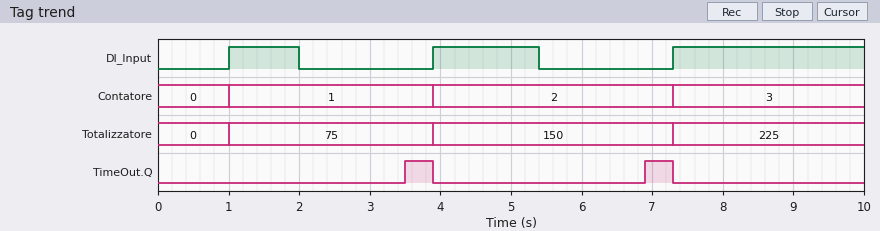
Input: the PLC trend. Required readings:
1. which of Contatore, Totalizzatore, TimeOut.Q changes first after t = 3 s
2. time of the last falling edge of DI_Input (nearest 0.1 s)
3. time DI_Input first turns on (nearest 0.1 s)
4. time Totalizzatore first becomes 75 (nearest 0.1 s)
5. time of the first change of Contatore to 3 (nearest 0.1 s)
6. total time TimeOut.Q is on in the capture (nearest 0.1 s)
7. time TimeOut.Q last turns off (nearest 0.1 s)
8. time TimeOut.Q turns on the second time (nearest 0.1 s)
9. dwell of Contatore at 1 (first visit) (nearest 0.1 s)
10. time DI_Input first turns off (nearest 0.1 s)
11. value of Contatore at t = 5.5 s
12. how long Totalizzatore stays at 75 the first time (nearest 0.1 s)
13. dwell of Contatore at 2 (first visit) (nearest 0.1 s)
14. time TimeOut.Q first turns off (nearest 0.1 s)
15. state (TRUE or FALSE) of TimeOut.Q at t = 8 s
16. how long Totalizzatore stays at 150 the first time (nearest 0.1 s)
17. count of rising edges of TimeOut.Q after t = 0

TimeOut.Q
5.4 s
1.0 s
1.0 s
7.3 s
0.8 s
7.3 s
6.9 s
2.9 s
2.0 s
2
2.9 s
3.4 s
3.9 s
FALSE
3.4 s
2
